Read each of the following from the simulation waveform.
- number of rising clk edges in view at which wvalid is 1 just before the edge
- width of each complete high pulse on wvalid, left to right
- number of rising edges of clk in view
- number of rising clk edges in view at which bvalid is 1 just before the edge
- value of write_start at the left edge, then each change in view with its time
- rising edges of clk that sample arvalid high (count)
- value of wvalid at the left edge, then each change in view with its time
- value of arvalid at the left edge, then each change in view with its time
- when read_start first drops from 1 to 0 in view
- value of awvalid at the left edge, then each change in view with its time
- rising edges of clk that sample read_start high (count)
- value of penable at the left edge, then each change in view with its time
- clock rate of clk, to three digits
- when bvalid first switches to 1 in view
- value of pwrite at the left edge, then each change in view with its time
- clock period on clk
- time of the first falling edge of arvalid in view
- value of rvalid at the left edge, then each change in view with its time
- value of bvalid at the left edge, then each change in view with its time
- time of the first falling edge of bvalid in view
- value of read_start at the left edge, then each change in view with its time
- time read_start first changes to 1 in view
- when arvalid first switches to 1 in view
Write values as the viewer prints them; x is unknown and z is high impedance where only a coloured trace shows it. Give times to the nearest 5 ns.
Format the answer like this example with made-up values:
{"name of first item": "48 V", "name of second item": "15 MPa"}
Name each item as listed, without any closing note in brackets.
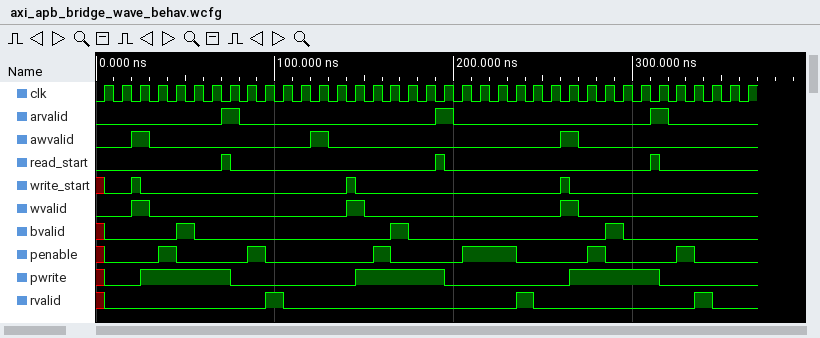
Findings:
{"number of rising clk edges in view at which wvalid is 1 just before the edge": "3", "width of each complete high pulse on wvalid, left to right": "10 ns, 10 ns, 10 ns", "number of rising edges of clk in view": "37", "number of rising clk edges in view at which bvalid is 1 just before the edge": "3", "value of write_start at the left edge, then each change in view with its time": "x, 0 at 5 ns, 1 at 20 ns, 0 at 25 ns, 1 at 140 ns, 0 at 145 ns, 1 at 260 ns, 0 at 265 ns", "rising edges of clk that sample arvalid high": "3", "value of wvalid at the left edge, then each change in view with its time": "0, 1 at 20 ns, 0 at 30 ns, 1 at 140 ns, 0 at 150 ns, 1 at 260 ns, 0 at 270 ns", "value of arvalid at the left edge, then each change in view with its time": "0, 1 at 70 ns, 0 at 80 ns, 1 at 190 ns, 0 at 200 ns, 1 at 310 ns, 0 at 320 ns", "when read_start first drops from 1 to 0 in view": "75 ns", "value of awvalid at the left edge, then each change in view with its time": "0, 1 at 20 ns, 0 at 30 ns, 1 at 120 ns, 0 at 130 ns, 1 at 260 ns, 0 at 270 ns", "rising edges of clk that sample read_start high": "3", "value of penable at the left edge, then each change in view with its time": "x, 0 at 5 ns, 1 at 35 ns, 0 at 45 ns, 1 at 85 ns, 0 at 95 ns, 1 at 155 ns, 0 at 165 ns, 1 at 205 ns, 0 at 235 ns, 1 at 275 ns, 0 at 285 ns, 1 at 325 ns, 0 at 335 ns", "clock rate of clk, to three digits": "100 MHz", "when bvalid first switches to 1 in view": "45 ns", "value of pwrite at the left edge, then each change in view with its time": "x, 0 at 5 ns, 1 at 25 ns, 0 at 75 ns, 1 at 145 ns, 0 at 195 ns, 1 at 265 ns, 0 at 315 ns", "clock period on clk": "10 ns", "time of the first falling edge of arvalid in view": "80 ns", "value of rvalid at the left edge, then each change in view with its time": "x, 0 at 5 ns, 1 at 95 ns, 0 at 105 ns, 1 at 235 ns, 0 at 245 ns, 1 at 335 ns, 0 at 345 ns", "value of bvalid at the left edge, then each change in view with its time": "x, 0 at 5 ns, 1 at 45 ns, 0 at 55 ns, 1 at 165 ns, 0 at 175 ns, 1 at 285 ns, 0 at 295 ns", "time of the first falling edge of bvalid in view": "55 ns", "value of read_start at the left edge, then each change in view with its time": "0, 1 at 70 ns, 0 at 75 ns, 1 at 190 ns, 0 at 195 ns, 1 at 310 ns, 0 at 315 ns", "time read_start first changes to 1 in view": "70 ns", "when arvalid first switches to 1 in view": "70 ns"}
